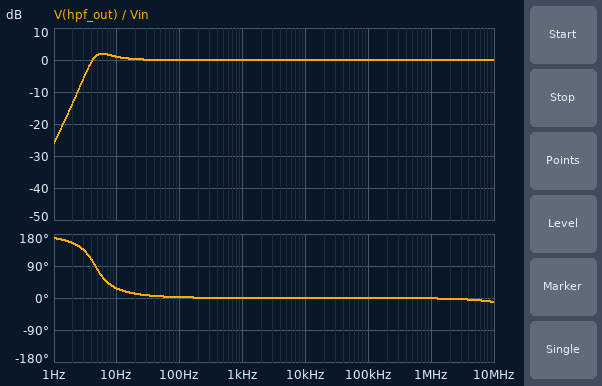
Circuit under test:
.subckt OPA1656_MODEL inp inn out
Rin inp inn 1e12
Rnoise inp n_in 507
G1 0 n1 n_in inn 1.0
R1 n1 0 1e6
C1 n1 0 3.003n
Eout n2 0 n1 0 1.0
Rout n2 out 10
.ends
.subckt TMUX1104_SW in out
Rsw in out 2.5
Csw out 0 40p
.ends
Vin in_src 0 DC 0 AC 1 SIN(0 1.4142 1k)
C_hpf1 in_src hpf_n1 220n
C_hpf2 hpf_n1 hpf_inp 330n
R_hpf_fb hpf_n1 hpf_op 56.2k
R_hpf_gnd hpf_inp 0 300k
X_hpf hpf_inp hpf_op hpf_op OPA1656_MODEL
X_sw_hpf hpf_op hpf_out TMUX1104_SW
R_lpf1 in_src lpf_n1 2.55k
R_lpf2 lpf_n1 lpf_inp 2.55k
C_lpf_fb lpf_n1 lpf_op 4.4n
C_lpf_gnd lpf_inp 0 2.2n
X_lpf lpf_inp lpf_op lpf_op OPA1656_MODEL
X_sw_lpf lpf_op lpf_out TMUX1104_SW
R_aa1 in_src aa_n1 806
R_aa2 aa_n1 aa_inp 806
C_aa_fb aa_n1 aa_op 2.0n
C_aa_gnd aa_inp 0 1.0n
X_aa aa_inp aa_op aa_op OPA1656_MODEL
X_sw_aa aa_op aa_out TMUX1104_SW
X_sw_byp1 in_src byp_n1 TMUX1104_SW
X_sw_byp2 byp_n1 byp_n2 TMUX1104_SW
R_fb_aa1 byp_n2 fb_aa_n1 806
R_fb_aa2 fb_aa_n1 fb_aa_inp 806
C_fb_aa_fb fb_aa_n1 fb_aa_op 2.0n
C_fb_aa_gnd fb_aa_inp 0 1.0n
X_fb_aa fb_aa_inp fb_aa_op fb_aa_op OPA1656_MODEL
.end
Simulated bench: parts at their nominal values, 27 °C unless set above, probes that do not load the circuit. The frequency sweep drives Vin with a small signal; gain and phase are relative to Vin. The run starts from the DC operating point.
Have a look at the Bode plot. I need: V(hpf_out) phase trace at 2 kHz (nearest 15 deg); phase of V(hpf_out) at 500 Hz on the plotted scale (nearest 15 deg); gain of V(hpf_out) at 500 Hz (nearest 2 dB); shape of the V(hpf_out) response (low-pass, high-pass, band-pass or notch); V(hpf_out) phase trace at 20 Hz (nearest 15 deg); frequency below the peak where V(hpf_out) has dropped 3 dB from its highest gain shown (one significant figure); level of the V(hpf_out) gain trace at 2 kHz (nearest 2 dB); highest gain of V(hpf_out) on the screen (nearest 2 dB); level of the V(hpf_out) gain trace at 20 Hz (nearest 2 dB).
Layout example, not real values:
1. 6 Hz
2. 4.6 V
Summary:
1. 0 deg
2. 0 deg
3. 0 dB
4. high-pass
5. 15 deg
6. 4 Hz
7. 0 dB
8. 2 dB
9. 0 dB
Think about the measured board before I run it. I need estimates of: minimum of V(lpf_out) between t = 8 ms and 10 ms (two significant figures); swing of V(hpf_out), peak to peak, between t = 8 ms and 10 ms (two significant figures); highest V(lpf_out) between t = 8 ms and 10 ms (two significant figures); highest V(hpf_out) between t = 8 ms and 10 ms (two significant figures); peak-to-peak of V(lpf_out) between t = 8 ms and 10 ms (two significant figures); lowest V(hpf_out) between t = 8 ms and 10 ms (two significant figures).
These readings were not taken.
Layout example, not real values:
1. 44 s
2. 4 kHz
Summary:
1. -1.4 V
2. 2.8 V
3. 1.4 V
4. 1.4 V
5. 2.8 V
6. -1.4 V
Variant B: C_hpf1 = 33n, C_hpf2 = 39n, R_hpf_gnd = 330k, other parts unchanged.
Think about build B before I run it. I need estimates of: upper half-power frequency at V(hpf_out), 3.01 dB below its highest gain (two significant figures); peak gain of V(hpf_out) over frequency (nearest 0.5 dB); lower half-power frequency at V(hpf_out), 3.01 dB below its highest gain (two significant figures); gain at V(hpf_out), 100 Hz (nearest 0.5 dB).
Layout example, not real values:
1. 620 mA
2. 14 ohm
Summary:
1. 23 MHz
2. 2.5 dB
3. 27 Hz
4. 0.5 dB
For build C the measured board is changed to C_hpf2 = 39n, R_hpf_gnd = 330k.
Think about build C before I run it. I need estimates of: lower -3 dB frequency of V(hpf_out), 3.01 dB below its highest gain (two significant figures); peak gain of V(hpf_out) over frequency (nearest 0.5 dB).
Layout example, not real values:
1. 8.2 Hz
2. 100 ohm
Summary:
1. 11 Hz
2. 0.5 dB
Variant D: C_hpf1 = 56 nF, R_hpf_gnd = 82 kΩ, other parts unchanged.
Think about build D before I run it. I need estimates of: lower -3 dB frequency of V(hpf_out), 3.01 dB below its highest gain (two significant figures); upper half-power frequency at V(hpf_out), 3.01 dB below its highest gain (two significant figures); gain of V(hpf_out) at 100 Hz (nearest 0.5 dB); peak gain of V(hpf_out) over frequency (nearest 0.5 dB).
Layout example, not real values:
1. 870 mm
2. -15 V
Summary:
1. 34 Hz
2. 60 MHz
3. -0.5 dB
4. 0 dB
